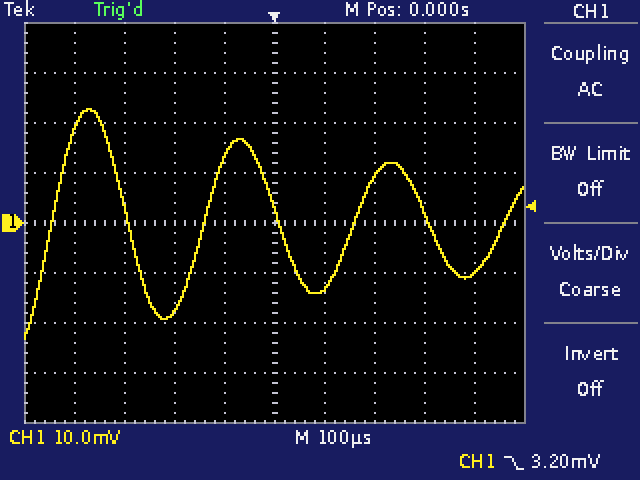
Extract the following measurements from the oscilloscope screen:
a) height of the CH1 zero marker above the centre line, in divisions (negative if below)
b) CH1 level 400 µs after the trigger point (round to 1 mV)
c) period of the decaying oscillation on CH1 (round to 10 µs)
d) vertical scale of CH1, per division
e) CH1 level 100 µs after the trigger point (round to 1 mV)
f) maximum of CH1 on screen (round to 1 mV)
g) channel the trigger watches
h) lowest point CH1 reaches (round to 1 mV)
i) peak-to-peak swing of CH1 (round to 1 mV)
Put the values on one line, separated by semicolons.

0.0 div; -10 mV; 300 µs; 10 mV; -13 mV; 23 mV; CH1; -23 mV; 46 mV
